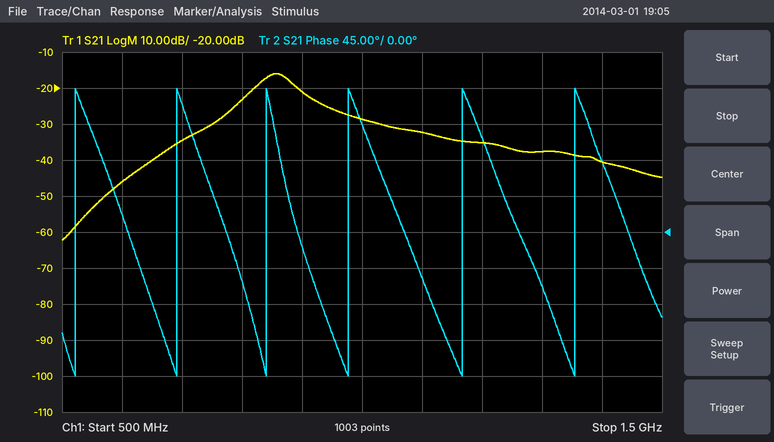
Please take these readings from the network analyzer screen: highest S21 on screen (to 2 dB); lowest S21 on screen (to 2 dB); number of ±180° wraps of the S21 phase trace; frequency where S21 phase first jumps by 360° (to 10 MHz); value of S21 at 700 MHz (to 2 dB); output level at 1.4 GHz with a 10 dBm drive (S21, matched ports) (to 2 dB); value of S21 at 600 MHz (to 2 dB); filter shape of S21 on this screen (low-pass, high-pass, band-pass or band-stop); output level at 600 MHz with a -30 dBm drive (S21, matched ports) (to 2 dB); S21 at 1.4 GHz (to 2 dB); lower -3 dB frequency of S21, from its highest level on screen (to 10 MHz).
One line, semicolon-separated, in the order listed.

-16 dB; -62 dB; 6; 520 MHz; -34 dB; -30 dBm; -46 dB; band-pass; -76 dBm; -40 dB; 830 MHz
